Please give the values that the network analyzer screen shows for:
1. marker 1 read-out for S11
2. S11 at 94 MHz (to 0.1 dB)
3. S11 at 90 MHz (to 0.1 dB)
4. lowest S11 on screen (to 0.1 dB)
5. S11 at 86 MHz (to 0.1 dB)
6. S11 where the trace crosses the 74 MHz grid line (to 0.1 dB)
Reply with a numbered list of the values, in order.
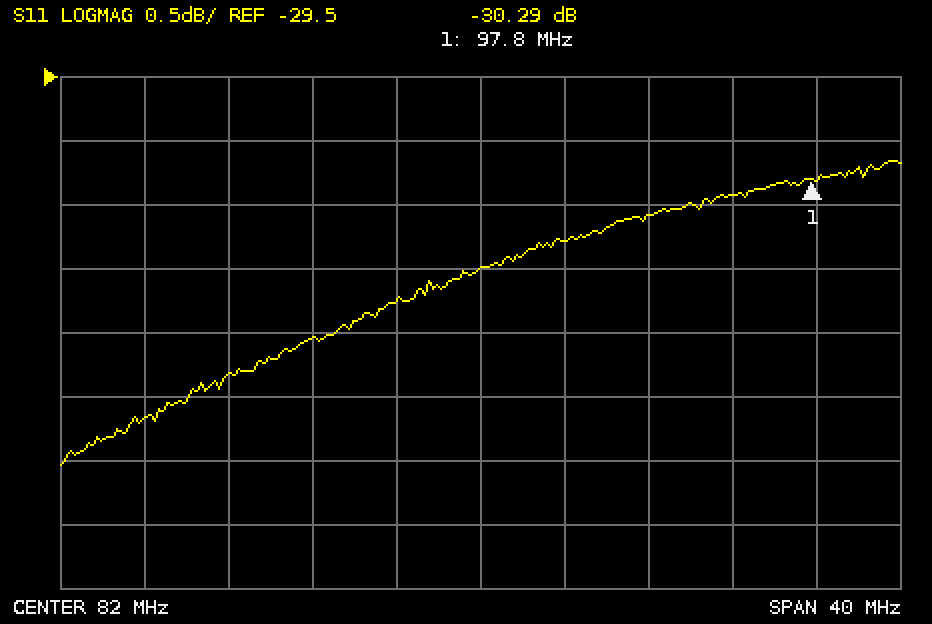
1. -30.29 dB
2. -30.4 dB
3. -30.6 dB
4. -32.5 dB
5. -30.8 dB
6. -31.5 dB
